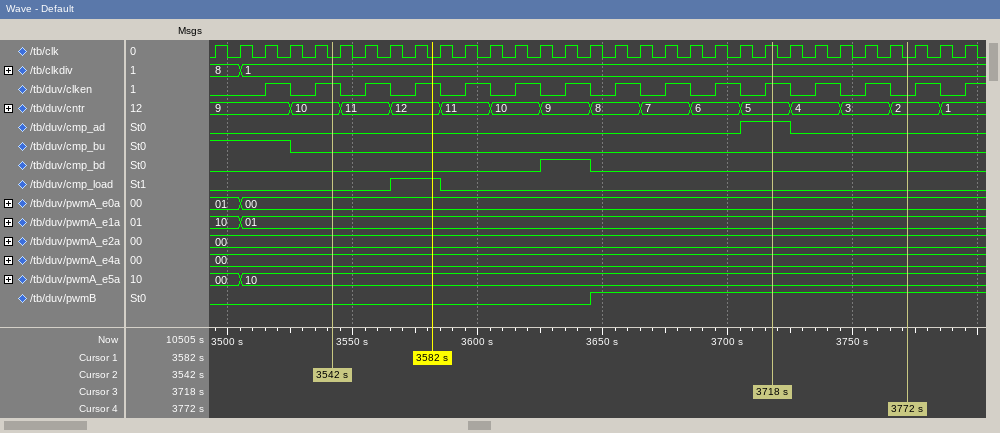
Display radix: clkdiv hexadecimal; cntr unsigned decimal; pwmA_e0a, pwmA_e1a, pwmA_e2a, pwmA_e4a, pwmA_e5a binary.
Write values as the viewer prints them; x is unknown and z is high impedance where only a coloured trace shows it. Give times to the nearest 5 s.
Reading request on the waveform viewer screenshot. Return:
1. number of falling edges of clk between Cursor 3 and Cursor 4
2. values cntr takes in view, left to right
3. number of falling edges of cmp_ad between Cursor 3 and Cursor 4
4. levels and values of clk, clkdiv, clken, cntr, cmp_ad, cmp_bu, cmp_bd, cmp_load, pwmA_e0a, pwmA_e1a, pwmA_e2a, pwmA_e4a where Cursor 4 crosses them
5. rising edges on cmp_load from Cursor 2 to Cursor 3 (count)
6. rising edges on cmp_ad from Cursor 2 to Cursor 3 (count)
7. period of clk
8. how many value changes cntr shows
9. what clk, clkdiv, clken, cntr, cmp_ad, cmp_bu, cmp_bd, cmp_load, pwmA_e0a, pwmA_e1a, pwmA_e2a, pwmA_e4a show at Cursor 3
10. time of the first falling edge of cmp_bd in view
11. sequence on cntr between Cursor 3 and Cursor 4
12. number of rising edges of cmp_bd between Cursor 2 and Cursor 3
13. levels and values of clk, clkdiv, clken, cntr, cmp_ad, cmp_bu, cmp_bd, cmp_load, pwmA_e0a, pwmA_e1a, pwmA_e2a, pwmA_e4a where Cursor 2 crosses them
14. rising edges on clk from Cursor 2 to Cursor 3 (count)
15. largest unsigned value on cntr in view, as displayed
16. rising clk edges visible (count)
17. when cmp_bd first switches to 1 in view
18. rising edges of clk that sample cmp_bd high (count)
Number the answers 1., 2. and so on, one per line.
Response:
1. 6
2. 9, 10, 11, 12, 11, 10, 9, 8, 7, 6, 5, 4, 3, 2, 1
3. 1
4. clk=0, clkdiv=1, clken=0, cntr=2, cmp_ad=0, cmp_bu=0, cmp_bd=0, cmp_load=0, pwmA_e0a=00, pwmA_e1a=01, pwmA_e2a=00, pwmA_e4a=00
5. 1
6. 1
7. 10 s
8. 14
9. clk=1, clkdiv=1, clken=1, cntr=5, cmp_ad=1, cmp_bu=0, cmp_bd=0, cmp_load=0, pwmA_e0a=00, pwmA_e1a=01, pwmA_e2a=00, pwmA_e4a=00
10. 3645 s
11. 5, 4, 3, 2
12. 1
13. clk=0, clkdiv=1, clken=1, cntr=10, cmp_ad=0, cmp_bu=0, cmp_bd=0, cmp_load=0, pwmA_e0a=00, pwmA_e1a=01, pwmA_e2a=00, pwmA_e4a=00
14. 18
15. 12
16. 31
17. 3625 s
18. 2
